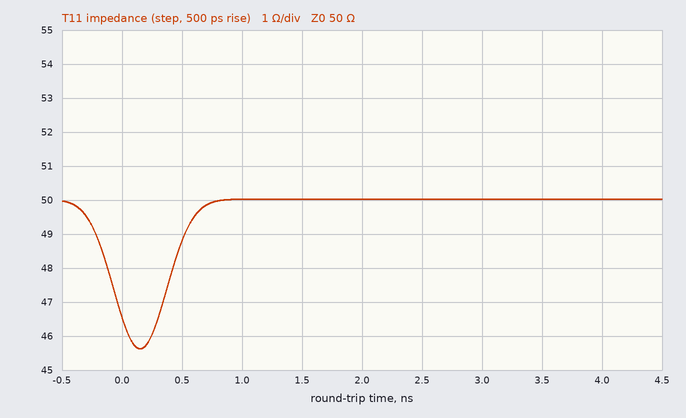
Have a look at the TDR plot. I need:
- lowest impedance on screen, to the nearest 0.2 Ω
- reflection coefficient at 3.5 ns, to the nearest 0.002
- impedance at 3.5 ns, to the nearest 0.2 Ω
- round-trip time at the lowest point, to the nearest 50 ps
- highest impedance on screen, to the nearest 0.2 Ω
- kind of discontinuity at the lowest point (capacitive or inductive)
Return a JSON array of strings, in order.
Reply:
["45.6 Ω", "0.000", "50.0 Ω", "150 ps", "50.0 Ω", "capacitive"]
